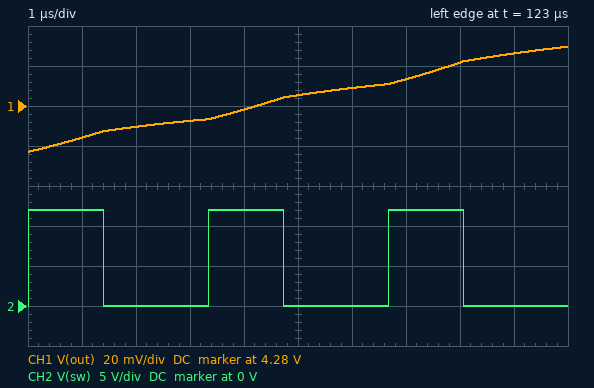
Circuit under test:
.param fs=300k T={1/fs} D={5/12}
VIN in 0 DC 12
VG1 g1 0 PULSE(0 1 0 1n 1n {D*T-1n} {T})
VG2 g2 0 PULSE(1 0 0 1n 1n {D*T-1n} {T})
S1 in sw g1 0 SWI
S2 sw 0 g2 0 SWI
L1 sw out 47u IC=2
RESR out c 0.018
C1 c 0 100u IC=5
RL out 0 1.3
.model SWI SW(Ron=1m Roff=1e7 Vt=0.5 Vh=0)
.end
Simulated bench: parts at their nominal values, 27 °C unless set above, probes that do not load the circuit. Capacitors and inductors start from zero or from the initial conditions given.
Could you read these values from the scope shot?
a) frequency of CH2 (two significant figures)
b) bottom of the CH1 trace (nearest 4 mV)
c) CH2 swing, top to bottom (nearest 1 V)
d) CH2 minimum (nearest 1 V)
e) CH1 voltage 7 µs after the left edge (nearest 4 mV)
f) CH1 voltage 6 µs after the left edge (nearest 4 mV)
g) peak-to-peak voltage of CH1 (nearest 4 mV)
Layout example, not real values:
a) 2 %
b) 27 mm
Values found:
a) 300 kHz
b) 4.256 V
c) 12 V
d) 0 V
e) 4.292 V
f) 4.288 V
g) 52 mV
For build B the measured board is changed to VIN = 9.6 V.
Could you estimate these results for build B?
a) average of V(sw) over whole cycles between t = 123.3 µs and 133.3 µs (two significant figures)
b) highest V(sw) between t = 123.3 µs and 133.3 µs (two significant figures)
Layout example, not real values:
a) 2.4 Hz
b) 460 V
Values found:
a) 4.0 V
b) 9.6 V
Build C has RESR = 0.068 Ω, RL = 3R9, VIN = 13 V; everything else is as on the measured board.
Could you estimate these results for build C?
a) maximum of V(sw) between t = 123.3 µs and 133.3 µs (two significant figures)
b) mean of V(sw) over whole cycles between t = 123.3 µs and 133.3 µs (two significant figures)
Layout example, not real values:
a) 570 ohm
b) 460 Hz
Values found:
a) 13 V
b) 5.4 V
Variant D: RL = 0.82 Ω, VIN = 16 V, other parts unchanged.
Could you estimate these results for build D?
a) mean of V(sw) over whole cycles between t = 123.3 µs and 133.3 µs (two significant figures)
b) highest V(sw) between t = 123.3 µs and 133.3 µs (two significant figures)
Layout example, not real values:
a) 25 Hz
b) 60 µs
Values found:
a) 6.7 V
b) 16 V
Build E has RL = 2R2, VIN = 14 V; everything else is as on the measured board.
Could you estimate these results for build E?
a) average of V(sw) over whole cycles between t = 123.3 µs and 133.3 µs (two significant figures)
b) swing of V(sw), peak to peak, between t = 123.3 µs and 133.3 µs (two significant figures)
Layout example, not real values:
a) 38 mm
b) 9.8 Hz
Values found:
a) 5.8 V
b) 14 V
